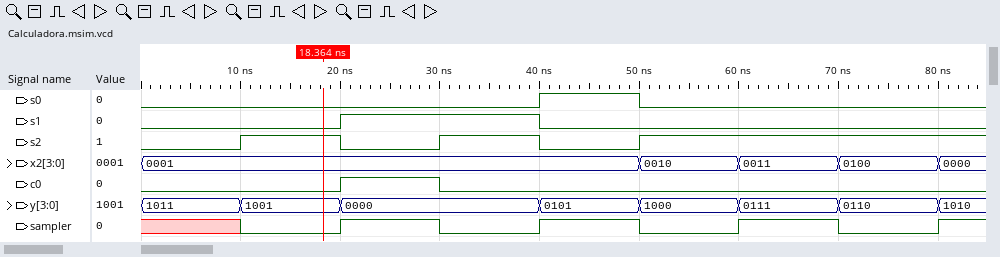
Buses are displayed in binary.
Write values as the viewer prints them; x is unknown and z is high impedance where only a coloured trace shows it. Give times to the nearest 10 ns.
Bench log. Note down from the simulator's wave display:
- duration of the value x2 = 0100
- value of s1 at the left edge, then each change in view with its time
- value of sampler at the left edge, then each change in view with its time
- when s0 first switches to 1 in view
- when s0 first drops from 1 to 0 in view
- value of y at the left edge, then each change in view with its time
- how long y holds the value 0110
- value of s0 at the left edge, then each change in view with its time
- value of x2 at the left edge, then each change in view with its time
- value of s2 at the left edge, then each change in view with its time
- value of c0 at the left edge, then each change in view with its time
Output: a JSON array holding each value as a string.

["10 ns", "0, 1 at 20 ns, 0 at 40 ns", "x, 0 at 10 ns, 1 at 20 ns, 0 at 30 ns, 1 at 40 ns, 0 at 50 ns, 1 at 60 ns, 0 at 70 ns, 1 at 80 ns", "40 ns", "50 ns", "1011, 1001 at 10 ns, 0000 at 20 ns, 0101 at 40 ns, 1000 at 50 ns, 0111 at 60 ns, 0110 at 70 ns, 1010 at 80 ns", "10 ns", "0, 1 at 40 ns, 0 at 50 ns", "0001, 0010 at 50 ns, 0011 at 60 ns, 0100 at 70 ns, 0000 at 80 ns", "0, 1 at 10 ns, 0 at 20 ns, 1 at 30 ns, 0 at 40 ns, 1 at 50 ns", "0, 1 at 20 ns, 0 at 30 ns"]
